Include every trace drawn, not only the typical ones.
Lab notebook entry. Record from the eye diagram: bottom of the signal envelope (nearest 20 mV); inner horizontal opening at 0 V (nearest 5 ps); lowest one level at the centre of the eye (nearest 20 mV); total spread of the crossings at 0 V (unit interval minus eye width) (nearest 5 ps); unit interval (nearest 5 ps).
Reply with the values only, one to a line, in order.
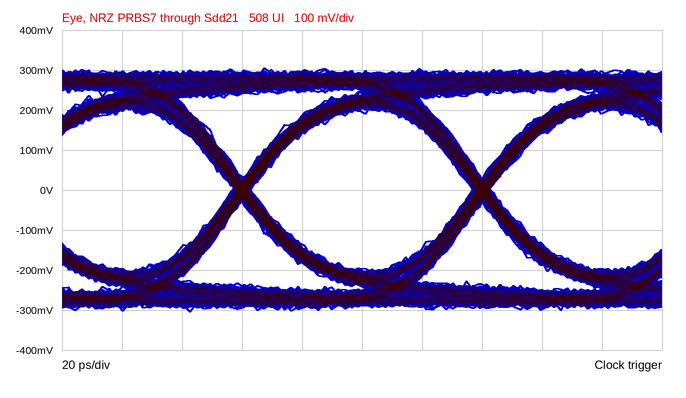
-300 mV
75 ps
200 mV
5 ps
80 ps
